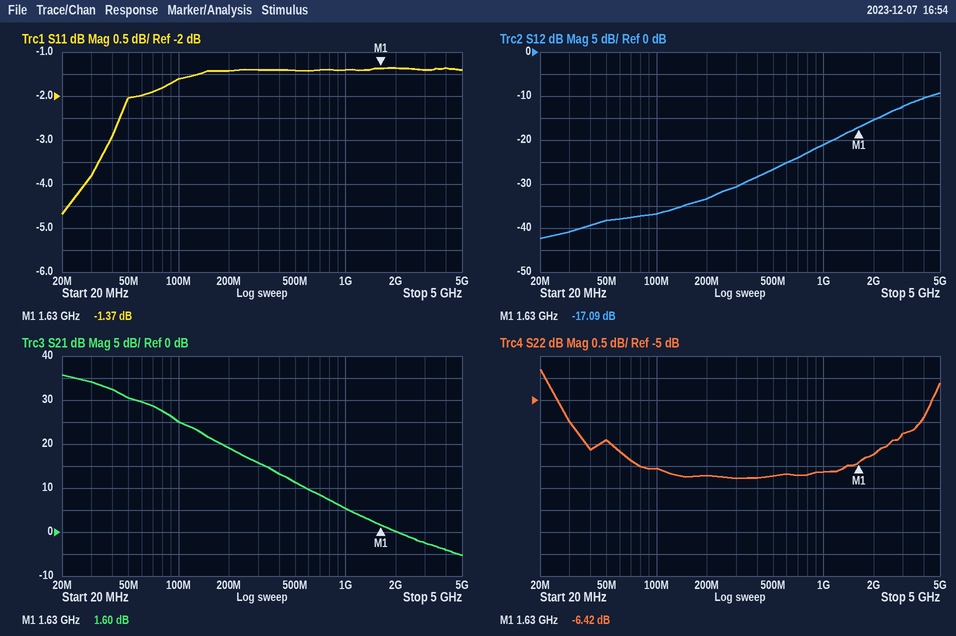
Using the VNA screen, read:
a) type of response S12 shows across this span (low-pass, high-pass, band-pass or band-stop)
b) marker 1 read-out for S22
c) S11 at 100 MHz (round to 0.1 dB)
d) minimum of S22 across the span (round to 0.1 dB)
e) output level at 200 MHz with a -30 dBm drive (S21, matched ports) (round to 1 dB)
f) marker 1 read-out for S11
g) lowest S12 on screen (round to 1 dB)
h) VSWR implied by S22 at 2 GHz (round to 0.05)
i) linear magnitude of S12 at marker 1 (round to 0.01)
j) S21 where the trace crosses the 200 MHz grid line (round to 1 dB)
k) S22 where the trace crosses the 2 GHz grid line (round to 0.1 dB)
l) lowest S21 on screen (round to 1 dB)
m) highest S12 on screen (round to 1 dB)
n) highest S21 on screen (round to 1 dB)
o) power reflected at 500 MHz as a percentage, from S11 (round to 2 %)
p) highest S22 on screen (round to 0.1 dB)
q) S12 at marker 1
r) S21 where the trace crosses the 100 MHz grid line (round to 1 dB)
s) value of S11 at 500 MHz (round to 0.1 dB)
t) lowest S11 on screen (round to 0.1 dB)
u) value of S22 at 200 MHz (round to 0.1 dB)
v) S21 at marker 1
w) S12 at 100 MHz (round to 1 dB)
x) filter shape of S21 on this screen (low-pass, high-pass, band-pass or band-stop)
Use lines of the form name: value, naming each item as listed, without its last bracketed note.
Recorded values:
type of response S12 shows across this span: high-pass
marker 1 read-out for S22: -6.42 dB
S11 at 100 MHz: -1.6 dB
minimum of S22 across the span: -6.8 dB
output level at 200 MHz with a -30 dBm drive (S21, matched ports): -11 dBm
marker 1 read-out for S11: -1.37 dB
lowest S12 on screen: -42 dB
VSWR implied by S22 at 2 GHz: 2.90
linear magnitude of S12 at marker 1: 0.14
S21 where the trace crosses the 200 MHz grid line: 19 dB
S22 where the trace crosses the 2 GHz grid line: -6.2 dB
lowest S21 on screen: -5 dB
highest S12 on screen: -9 dB
highest S21 on screen: 36 dB
power reflected at 500 MHz as a percentage, from S11: 72 %
highest S22 on screen: -4.3 dB
S12 at marker 1: -17.09 dB
S21 where the trace crosses the 100 MHz grid line: 25 dB
value of S11 at 500 MHz: -1.4 dB
lowest S11 on screen: -4.7 dB
value of S22 at 200 MHz: -6.7 dB
S21 at marker 1: 1.60 dB
S12 at 100 MHz: -37 dB
filter shape of S21 on this screen: low-pass
